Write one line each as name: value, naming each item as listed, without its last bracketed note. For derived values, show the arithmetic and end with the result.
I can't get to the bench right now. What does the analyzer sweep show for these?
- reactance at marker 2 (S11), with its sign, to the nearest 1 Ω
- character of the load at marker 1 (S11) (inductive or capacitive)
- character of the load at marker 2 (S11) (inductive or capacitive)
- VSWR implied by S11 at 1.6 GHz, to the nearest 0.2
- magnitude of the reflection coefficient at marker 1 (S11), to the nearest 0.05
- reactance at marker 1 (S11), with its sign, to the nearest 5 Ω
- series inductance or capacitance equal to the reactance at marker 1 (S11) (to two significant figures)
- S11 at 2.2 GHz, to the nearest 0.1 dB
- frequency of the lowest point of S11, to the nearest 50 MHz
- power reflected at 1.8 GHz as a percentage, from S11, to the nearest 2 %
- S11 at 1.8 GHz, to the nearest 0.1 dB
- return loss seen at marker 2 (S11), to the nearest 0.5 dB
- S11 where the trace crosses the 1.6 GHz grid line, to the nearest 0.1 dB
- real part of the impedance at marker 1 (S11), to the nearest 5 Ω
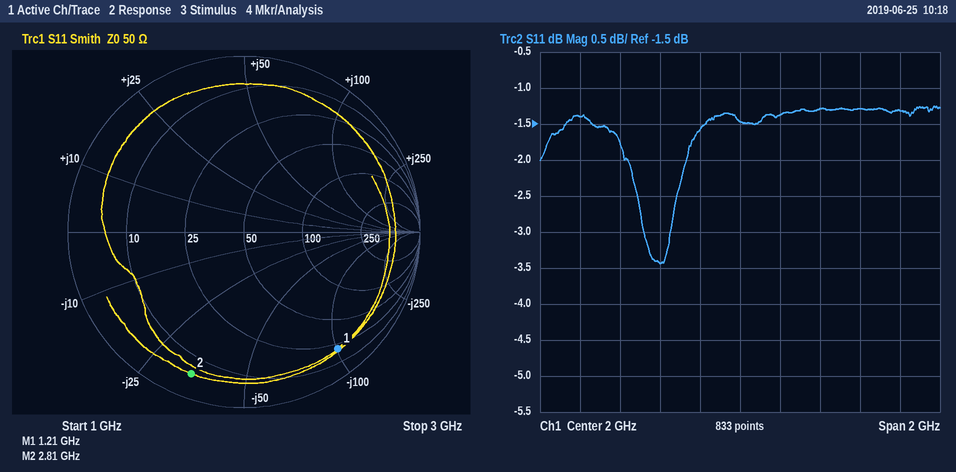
reactance at marker 2 (S11), with its sign, to the nearest 1 Ω: -34 Ω
character of the load at marker 1 (S11): capacitive
character of the load at marker 2 (S11): capacitive
VSWR implied by S11 at 1.6 GHz, to the nearest 0.2: |Γ| = 10^(-3.4/20) = 0.6761; VSWR = (1 + 0.6761)/(1 − 0.6761) ≈ 5.2
magnitude of the reflection coefficient at marker 1 (S11), to the nearest 0.05: 0.85
reactance at marker 1 (S11), with its sign, to the nearest 5 Ω: -100 Ω
series inductance or capacitance equal to the reactance at marker 1 (S11): C = 1/(2π × 1.21 GHz × 100 Ω) ≈ 1.3 pF
S11 at 2.2 GHz, to the nearest 0.1 dB: -1.4 dB
frequency of the lowest point of S11, to the nearest 50 MHz: 1.60 GHz
power reflected at 1.8 GHz as a percentage, from S11, to the nearest 2 %: 10^(-1.6/10) ≈ 69.2 %, so 70 % to the nearest 2 %
S11 at 1.8 GHz, to the nearest 0.1 dB: -1.6 dB
return loss seen at marker 2 (S11), to the nearest 0.5 dB: 1.5 dB
S11 where the trace crosses the 1.6 GHz grid line, to the nearest 0.1 dB: -3.4 dB
real part of the impedance at marker 1 (S11), to the nearest 5 Ω: 20 Ω
